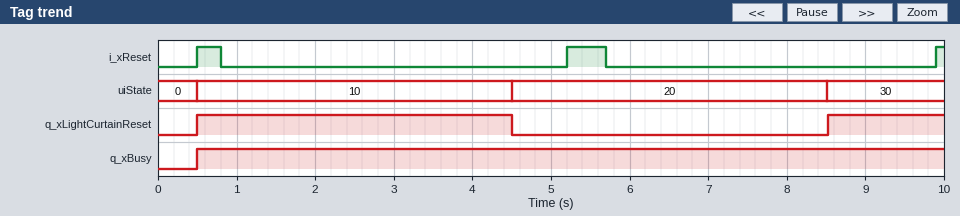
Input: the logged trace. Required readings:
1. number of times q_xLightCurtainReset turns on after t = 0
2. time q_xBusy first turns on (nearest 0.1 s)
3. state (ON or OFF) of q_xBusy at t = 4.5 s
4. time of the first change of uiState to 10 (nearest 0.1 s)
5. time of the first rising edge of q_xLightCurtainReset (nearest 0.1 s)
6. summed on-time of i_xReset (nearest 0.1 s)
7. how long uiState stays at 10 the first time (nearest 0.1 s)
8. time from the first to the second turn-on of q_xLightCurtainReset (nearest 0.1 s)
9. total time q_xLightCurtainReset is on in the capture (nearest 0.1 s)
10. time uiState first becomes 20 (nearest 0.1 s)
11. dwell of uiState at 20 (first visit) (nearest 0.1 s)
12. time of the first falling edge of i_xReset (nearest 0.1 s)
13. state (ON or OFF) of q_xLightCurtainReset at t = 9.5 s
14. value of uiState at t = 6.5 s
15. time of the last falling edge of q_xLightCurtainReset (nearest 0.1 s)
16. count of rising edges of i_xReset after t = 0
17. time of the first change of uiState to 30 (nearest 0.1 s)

2
0.5 s
ON
0.5 s
0.5 s
0.9 s
4.0 s
8.0 s
5.5 s
4.5 s
4.0 s
0.8 s
ON
20
4.5 s
3
8.5 s
